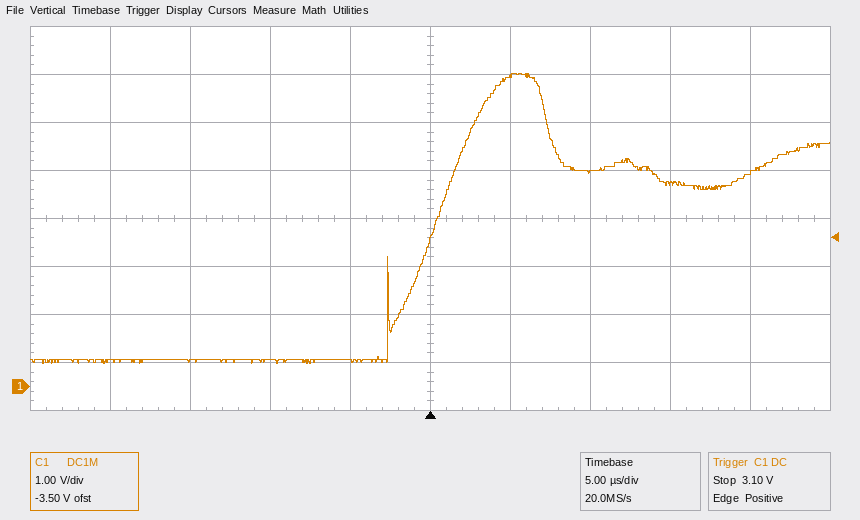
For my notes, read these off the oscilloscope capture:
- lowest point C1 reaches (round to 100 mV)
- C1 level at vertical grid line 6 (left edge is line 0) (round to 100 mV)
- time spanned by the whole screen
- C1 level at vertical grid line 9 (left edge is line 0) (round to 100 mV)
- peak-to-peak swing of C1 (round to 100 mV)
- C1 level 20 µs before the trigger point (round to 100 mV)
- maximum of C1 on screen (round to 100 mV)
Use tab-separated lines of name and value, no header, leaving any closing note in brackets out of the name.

lowest point C1 reaches	500 mV
C1 level at vertical grid line 6 (left edge is line 0)	6.5 V
time spanned by the whole screen	50 µs
C1 level at vertical grid line 9 (left edge is line 0)	4.5 V
peak-to-peak swing of C1	6.0 V
C1 level 20 µs before the trigger point	500 mV
maximum of C1 on screen	6.5 V
